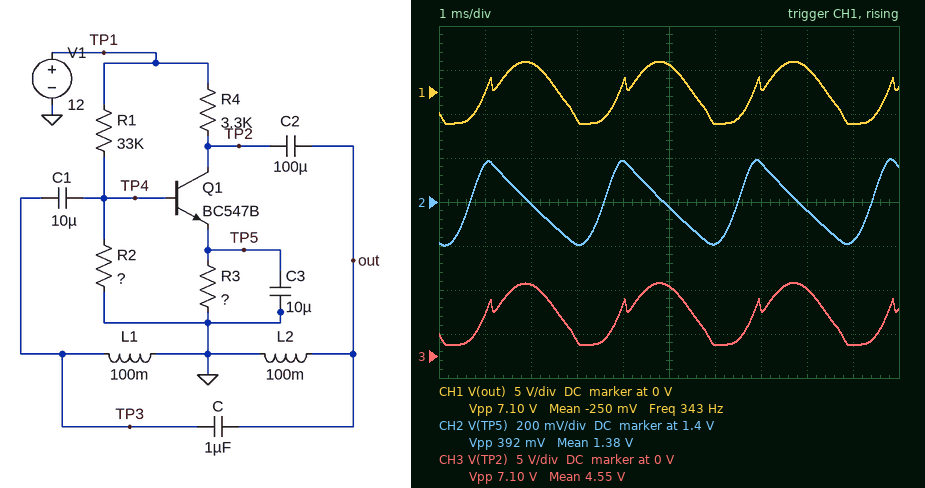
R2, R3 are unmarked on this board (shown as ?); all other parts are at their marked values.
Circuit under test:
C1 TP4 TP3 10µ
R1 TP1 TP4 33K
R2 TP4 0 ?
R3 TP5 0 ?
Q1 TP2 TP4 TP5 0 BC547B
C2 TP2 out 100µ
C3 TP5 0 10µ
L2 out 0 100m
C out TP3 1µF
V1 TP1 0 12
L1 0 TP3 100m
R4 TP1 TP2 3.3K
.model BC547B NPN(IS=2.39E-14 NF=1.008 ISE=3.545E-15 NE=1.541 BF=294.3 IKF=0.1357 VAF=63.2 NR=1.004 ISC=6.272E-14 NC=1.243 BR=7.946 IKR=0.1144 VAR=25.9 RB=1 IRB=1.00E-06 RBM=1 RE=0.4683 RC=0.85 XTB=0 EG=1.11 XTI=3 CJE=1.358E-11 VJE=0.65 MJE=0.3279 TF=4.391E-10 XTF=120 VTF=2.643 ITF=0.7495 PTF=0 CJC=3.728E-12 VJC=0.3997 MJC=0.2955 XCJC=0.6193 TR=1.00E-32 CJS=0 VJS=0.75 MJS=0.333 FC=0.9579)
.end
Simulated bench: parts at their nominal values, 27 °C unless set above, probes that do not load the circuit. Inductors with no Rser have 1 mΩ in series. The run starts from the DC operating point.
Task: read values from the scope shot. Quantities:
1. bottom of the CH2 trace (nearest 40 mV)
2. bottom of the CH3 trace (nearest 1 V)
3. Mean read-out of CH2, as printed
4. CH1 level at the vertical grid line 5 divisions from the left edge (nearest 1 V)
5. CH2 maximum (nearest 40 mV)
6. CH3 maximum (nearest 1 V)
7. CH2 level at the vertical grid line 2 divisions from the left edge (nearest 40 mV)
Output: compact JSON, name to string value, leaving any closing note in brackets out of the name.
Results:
{"bottom of the CH2 trace": "1.20 V", "bottom of the CH3 trace": "1 V", "Mean read-out of CH2, as printed": "1.38 V", "CH1 level at the vertical grid line 5 divisions from the left edge": "3 V", "CH2 maximum": "1.60 V", "CH3 maximum": "8 V", "CH2 level at the vertical grid line 2 divisions from the left edge": "1.40 V"}
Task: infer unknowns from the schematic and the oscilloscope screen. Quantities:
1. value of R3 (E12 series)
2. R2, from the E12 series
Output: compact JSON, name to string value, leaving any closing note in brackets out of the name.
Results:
{"value of R3": "680 Ω", "R2, from the E12 series": "8.2 kΩ"}
